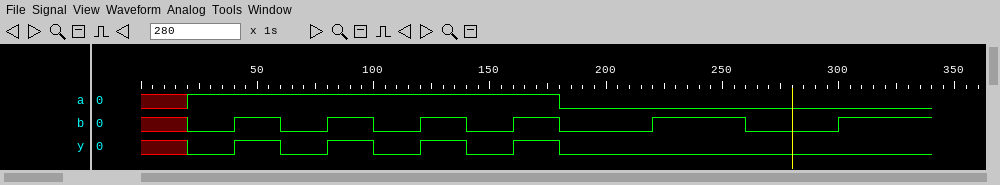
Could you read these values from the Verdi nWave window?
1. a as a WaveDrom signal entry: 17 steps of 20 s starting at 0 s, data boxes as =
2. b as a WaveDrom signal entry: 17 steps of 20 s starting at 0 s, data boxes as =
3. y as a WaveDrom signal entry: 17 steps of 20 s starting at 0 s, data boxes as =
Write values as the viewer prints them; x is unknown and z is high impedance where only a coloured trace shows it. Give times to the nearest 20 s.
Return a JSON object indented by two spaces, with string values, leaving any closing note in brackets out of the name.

{
  "a as a WaveDrom signal entry: 17 steps of 20 s starting at 0 s, data boxes as =": "{name: 'a', wave: 'x1.......0.......'}",
  "b as a WaveDrom signal entry: 17 steps of 20 s starting at 0 s, data boxes as =": "{name: 'b', wave: 'x010101010.1.0.1.'}",
  "y as a WaveDrom signal entry: 17 steps of 20 s starting at 0 s, data boxes as =": "{name: 'y', wave: 'x010101010.......'}"
}
